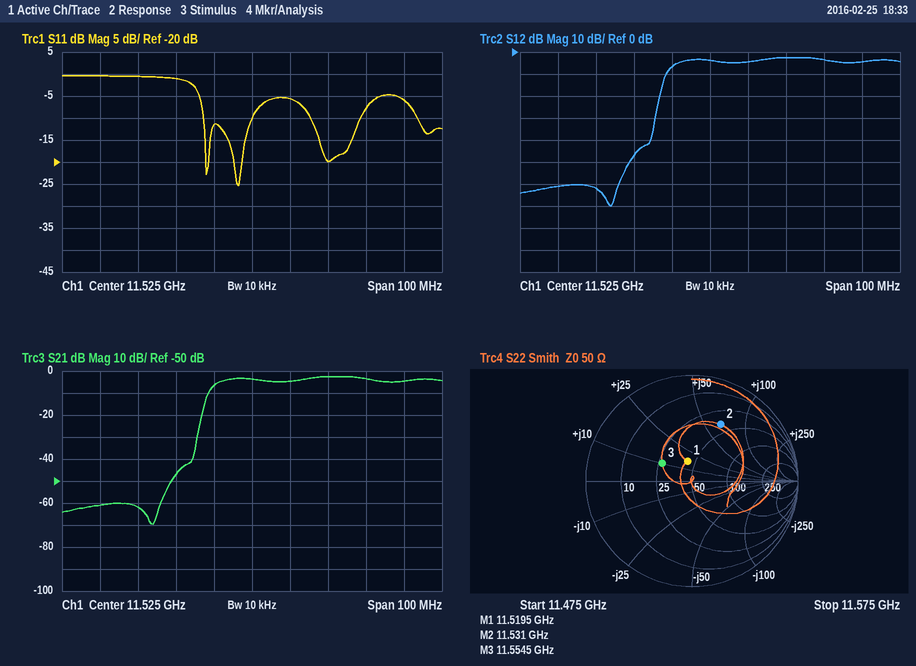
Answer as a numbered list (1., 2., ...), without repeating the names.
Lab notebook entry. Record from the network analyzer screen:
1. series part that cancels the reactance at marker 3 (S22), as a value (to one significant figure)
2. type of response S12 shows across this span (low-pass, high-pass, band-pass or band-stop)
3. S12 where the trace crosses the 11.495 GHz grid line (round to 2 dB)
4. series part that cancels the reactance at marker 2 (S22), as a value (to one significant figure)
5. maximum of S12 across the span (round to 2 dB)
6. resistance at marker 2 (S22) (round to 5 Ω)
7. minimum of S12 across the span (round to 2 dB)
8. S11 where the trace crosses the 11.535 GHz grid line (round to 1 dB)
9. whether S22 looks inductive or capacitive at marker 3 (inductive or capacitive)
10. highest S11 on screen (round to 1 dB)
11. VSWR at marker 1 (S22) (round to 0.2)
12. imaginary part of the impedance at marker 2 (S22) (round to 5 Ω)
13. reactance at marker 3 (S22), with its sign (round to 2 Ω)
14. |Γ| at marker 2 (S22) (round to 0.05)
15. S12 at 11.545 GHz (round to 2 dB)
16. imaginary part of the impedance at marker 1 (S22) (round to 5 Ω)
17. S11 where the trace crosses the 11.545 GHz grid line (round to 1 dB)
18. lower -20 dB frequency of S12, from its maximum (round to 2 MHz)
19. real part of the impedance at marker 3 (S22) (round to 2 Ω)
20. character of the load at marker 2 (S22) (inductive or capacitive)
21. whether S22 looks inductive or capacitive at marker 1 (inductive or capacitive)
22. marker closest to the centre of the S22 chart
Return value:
1. 1 pF
2. high-pass
3. -62 dB
4. 200 fF
5. -2 dB
6. 40 Ω
7. -70 dB
8. -6 dB
9. inductive
10. 0 dB
11. 1.4
12. +65 Ω
13. +10 Ω
14. 0.60
15. -2 dB
16. +15 Ω
17. -20 dB
18. 11.512 GHz
19. 26 Ω
20. inductive
21. inductive
22. marker 1
